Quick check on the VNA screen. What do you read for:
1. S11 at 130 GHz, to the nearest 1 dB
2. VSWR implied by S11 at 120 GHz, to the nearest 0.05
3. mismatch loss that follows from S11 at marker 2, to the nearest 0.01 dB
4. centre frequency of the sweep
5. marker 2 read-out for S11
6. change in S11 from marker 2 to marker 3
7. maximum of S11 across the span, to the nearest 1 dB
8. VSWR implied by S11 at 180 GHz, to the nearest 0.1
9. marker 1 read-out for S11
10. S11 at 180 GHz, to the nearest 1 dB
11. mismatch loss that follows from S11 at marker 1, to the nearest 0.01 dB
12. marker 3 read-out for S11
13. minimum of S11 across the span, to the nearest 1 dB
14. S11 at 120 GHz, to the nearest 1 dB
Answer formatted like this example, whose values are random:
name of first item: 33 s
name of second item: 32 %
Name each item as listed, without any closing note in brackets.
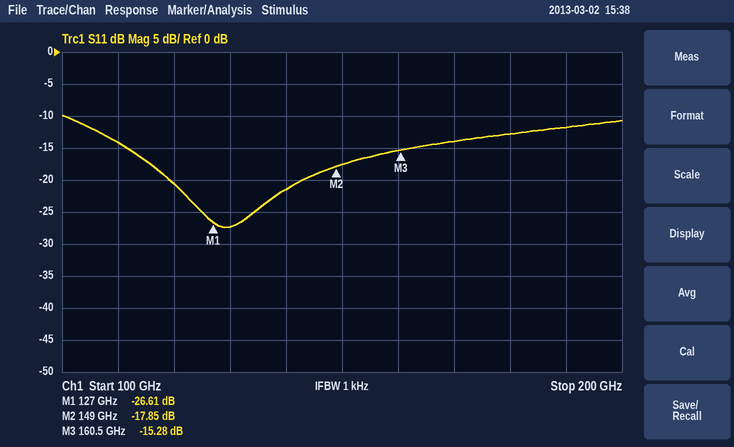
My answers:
S11 at 130 GHz, to the nearest 1 dB: -27 dB
VSWR implied by S11 at 120 GHz, to the nearest 0.05: 1.20
mismatch loss that follows from S11 at marker 2, to the nearest 0.01 dB: 0.07 dB
centre frequency of the sweep: 150 GHz
marker 2 read-out for S11: -17.85 dB
change in S11 from marker 2 to marker 3: 2.57 dB
maximum of S11 across the span, to the nearest 1 dB: -10 dB
VSWR implied by S11 at 180 GHz, to the nearest 0.1: 1.6
marker 1 read-out for S11: -26.61 dB
S11 at 180 GHz, to the nearest 1 dB: -13 dB
mismatch loss that follows from S11 at marker 1, to the nearest 0.01 dB: 0.01 dB
marker 3 read-out for S11: -15.28 dB
minimum of S11 across the span, to the nearest 1 dB: -27 dB
S11 at 120 GHz, to the nearest 1 dB: -21 dB
